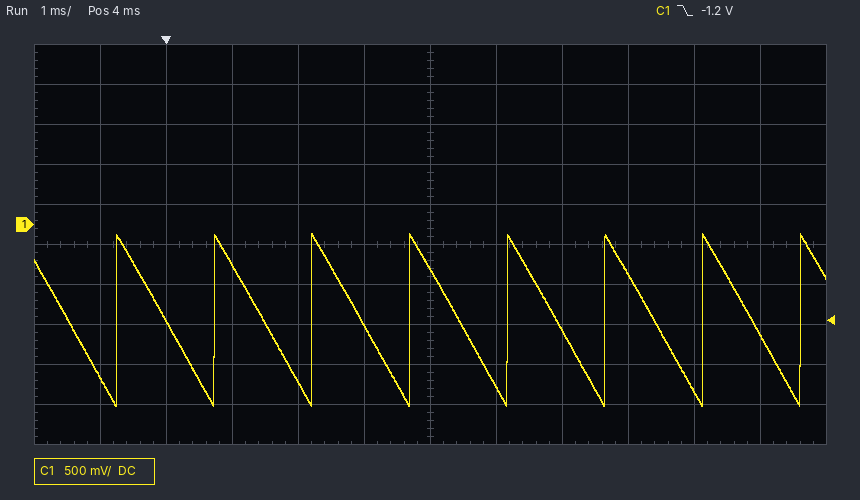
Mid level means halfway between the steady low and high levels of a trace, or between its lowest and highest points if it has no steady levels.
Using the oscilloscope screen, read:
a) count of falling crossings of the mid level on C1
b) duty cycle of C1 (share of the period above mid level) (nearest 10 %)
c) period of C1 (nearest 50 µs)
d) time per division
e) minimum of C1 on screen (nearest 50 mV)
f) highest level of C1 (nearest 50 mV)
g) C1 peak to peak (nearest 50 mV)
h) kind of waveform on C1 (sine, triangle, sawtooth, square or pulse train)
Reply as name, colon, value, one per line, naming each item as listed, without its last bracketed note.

count of falling crossings of the mid level on C1: 8
duty cycle of C1 (share of the period above mid level): 50 %
period of C1: 1.50 ms
time per division: 1 ms
minimum of C1 on screen: -2.25 V
highest level of C1: -100 mV
C1 peak to peak: 2.15 V
kind of waveform on C1: sawtooth
